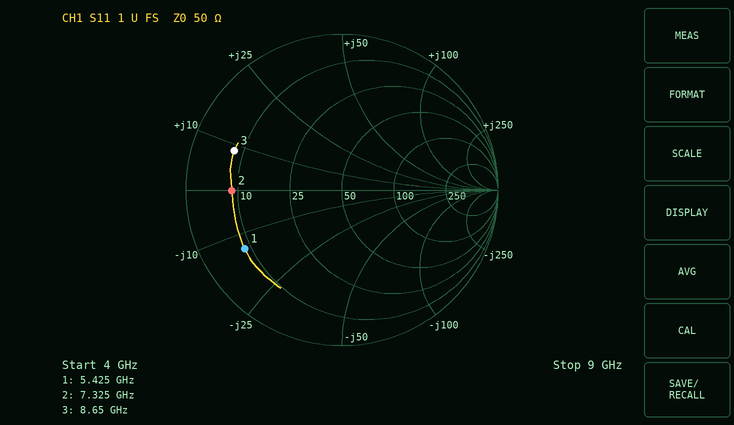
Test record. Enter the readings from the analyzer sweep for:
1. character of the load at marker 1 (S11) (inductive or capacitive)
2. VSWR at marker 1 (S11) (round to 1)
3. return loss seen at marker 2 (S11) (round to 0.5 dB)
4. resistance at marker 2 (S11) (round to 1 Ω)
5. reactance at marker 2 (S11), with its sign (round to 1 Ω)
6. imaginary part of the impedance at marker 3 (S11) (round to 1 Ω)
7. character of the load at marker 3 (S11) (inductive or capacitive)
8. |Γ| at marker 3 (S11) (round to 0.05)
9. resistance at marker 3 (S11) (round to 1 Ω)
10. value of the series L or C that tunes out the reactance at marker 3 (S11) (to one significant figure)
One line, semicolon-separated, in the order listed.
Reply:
capacitive; 6; 3.0 dB; 9 Ω; 0 Ω; +9 Ω; inductive; 0.75; 8 Ω; 2 pF
